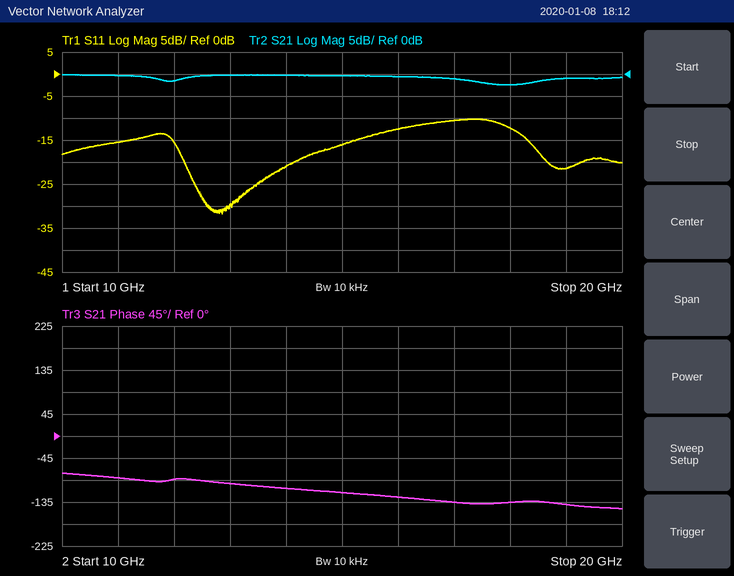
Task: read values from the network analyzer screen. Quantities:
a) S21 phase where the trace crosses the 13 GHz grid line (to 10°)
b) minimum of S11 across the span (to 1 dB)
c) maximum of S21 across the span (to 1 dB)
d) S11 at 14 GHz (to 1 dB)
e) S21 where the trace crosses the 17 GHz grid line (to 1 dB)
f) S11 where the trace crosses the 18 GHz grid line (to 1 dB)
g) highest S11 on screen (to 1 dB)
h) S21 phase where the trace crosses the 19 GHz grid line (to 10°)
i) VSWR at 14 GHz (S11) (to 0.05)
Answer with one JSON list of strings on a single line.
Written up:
["-100°", "-32 dB", "0 dB", "-21 dB", "-1 dB", "-12 dB", "-10 dB", "-140°", "1.20"]
